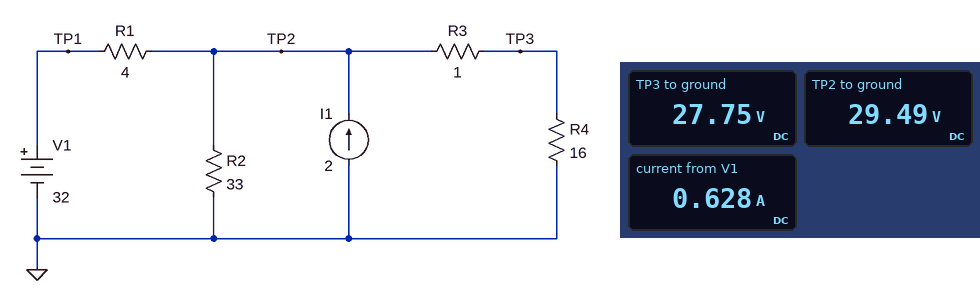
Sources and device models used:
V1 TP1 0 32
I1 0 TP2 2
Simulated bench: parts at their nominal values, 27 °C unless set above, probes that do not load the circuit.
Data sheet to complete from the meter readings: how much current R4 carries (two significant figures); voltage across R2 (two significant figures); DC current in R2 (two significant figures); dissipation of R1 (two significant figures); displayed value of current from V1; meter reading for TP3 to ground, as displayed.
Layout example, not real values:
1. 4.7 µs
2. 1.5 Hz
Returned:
1. 1.7 A
2. 29 V
3. 890 mA
4. 1.6 W
5. 0.628 A
6. 27.75 V
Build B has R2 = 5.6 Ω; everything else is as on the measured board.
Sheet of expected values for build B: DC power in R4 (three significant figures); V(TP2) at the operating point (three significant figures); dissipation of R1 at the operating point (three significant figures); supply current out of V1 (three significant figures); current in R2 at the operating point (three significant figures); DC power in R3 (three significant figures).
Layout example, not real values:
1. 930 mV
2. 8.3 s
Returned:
1. 23.3 W
2. 20.5 V
3. 33.0 W
4. 2.87 A
5. 3.66 A
6. 1.46 W
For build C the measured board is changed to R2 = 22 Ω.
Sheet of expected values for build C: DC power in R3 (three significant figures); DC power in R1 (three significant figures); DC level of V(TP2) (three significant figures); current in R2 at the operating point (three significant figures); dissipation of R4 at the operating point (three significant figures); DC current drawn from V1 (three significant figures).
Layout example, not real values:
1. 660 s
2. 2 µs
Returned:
1. 2.76 W
2. 3.56 W
3. 28.2 V
4. 1.28 A
5. 44.1 W
6. 943 mA
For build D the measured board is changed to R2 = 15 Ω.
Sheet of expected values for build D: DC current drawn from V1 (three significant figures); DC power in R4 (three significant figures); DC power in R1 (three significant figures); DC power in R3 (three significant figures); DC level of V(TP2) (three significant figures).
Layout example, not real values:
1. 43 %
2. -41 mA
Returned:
1. 1.34 A
2. 39.3 W
3. 7.20 W
4. 2.45 W
5. 26.6 V
